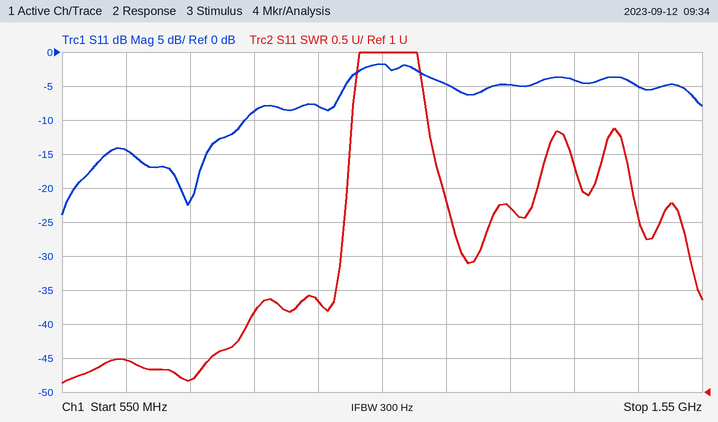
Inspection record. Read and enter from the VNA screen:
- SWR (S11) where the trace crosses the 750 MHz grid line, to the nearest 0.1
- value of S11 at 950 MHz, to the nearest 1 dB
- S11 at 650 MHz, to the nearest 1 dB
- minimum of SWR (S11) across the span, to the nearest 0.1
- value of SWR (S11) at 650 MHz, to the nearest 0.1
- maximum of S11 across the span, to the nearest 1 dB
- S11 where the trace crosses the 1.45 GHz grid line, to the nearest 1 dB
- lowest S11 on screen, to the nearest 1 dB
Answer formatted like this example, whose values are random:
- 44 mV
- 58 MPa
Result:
- 1.2
- -8 dB
- -14 dB
- 1.1
- 1.5
- -2 dB
- -5 dB
- -24 dB
